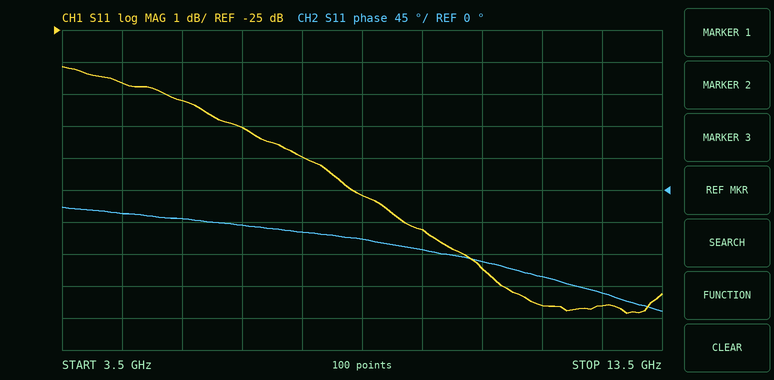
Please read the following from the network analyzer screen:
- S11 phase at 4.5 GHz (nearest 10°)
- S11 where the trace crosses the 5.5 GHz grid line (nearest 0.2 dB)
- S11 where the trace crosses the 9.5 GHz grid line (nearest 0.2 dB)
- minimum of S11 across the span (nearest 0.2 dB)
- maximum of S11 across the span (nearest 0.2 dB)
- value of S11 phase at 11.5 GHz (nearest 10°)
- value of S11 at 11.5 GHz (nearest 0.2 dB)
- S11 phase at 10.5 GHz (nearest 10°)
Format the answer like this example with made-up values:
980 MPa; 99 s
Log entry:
-30°; -27.2 dB; -31.2 dB; -33.8 dB; -26.2 dB; -120°; -33.6 dB; -100°
